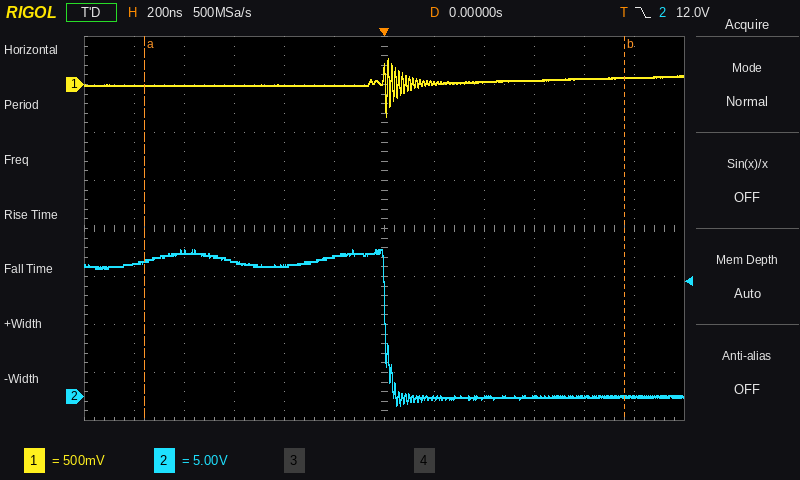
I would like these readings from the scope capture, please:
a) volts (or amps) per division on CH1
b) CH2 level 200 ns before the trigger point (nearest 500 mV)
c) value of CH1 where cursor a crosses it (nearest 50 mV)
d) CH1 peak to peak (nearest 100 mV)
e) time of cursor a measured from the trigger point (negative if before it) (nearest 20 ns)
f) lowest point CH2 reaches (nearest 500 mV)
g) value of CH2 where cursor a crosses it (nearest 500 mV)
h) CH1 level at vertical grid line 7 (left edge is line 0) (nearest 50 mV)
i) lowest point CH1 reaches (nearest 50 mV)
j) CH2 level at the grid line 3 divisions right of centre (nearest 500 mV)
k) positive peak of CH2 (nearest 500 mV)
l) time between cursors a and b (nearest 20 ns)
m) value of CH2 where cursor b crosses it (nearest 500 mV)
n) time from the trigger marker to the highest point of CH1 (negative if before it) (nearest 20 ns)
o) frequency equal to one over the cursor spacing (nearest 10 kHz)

500 mV
14.5 V
0 mV
600 mV
-960 ns
-1.0 V
14.0 V
0 mV
-350 mV
0.0 V
15.5 V
1.92 µs
0.0 V
+20 ns
520 kHz
